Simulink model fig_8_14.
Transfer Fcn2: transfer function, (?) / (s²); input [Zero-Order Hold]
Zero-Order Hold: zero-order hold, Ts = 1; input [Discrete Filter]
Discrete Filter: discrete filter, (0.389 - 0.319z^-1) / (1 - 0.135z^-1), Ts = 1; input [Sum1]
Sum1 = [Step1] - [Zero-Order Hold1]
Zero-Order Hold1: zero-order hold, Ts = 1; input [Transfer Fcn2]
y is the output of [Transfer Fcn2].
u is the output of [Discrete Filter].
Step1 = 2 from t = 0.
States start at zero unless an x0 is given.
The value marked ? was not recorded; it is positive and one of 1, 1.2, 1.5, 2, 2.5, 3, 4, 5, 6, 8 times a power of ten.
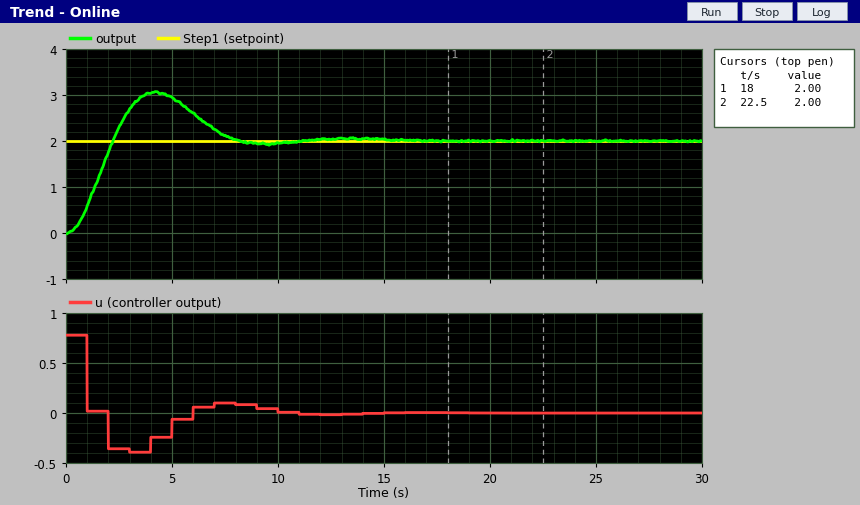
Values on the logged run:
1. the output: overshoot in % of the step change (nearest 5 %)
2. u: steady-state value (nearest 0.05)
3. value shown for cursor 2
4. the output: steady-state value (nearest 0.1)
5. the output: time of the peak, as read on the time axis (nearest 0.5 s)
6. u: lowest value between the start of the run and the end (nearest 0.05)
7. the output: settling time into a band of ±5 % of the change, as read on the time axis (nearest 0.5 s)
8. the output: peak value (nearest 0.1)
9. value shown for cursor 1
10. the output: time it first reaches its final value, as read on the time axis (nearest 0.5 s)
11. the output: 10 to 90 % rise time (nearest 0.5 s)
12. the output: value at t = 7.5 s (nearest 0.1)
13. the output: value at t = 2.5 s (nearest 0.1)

55 %
0.00
2.00
2.0
4.0 s
-0.40
7.5 s
3.1
2.00
2.0 s
1.5 s
2.1
2.3
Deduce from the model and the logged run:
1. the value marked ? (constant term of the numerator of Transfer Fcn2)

1.5
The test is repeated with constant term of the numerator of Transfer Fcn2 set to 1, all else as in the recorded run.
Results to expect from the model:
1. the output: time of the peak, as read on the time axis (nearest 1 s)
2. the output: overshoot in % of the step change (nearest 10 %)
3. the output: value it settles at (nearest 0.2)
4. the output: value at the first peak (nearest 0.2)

6 s
40 %
2.0
2.8
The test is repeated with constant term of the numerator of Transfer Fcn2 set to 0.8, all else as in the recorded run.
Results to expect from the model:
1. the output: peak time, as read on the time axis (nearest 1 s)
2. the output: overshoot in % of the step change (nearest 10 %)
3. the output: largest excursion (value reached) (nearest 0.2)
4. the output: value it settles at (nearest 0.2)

7 s
40 %
2.8
2.0
